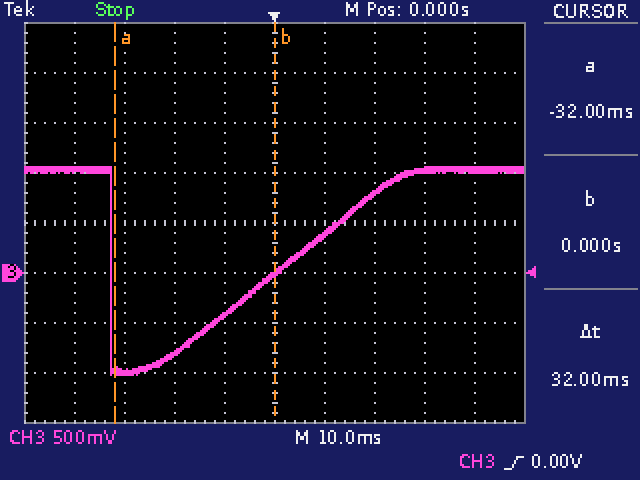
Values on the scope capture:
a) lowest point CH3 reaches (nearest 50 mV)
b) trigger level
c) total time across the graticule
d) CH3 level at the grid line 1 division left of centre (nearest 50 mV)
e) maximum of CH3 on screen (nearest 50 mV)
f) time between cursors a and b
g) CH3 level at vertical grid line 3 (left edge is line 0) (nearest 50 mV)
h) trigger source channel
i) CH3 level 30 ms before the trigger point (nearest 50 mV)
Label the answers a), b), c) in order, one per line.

a) -1.00 V
b) 0.00 V
c) 100 ms
d) -400 mV
e) 1.05 V
f) 32 ms
g) -800 mV
h) CH3
i) -1.00 V
